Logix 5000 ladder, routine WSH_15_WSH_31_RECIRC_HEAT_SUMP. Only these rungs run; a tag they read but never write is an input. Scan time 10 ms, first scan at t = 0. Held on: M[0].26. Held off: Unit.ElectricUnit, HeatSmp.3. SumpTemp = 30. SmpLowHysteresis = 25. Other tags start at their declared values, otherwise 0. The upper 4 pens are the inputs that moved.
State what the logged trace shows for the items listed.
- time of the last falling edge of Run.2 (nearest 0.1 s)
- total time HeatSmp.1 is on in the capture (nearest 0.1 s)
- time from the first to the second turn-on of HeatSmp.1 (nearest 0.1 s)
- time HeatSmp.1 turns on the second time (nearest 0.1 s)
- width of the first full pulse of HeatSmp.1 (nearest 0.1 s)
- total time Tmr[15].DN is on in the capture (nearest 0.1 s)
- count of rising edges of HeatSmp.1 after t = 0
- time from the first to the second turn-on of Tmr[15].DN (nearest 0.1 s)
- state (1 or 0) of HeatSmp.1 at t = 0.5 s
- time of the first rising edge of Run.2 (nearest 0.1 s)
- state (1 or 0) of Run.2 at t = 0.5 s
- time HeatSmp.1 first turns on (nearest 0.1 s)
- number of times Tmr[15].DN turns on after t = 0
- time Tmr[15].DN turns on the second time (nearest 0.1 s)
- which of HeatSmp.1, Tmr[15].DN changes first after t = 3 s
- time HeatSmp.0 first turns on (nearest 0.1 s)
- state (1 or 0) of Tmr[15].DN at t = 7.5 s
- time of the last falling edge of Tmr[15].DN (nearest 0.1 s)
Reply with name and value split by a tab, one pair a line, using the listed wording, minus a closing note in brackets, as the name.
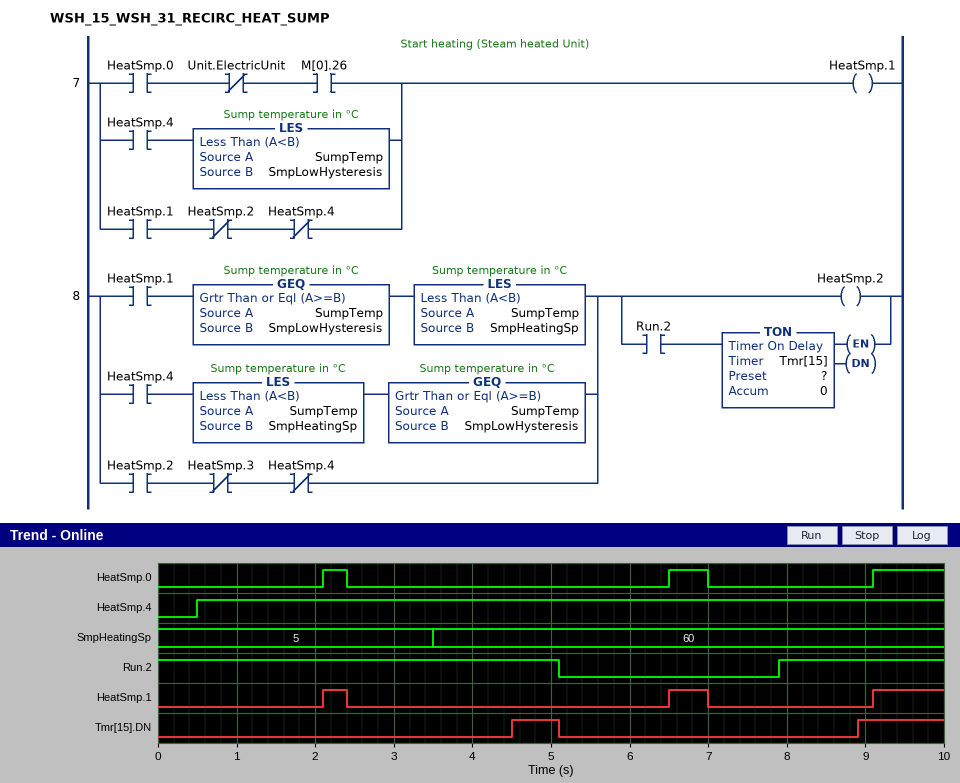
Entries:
time of the last falling edge of Run.2	5.1 s
total time HeatSmp.1 is on in the capture	1.7 s
time from the first to the second turn-on of HeatSmp.1	4.4 s
time HeatSmp.1 turns on the second time	6.5 s
width of the first full pulse of HeatSmp.1	0.3 s
total time Tmr[15].DN is on in the capture	1.7 s
count of rising edges of HeatSmp.1 after t = 0	3
time from the first to the second turn-on of Tmr[15].DN	4.4 s
state (1 or 0) of HeatSmp.1 at t = 0.5 s	0
time of the first rising edge of Run.2	7.9 s
state (1 or 0) of Run.2 at t = 0.5 s	1
time HeatSmp.1 first turns on	2.1 s
number of times Tmr[15].DN turns on after t = 0	2
time Tmr[15].DN turns on the second time	8.9 s
which of HeatSmp.1, Tmr[15].DN changes first after t = 3 s	Tmr[15].DN
time HeatSmp.0 first turns on	2.1 s
state (1 or 0) of Tmr[15].DN at t = 7.5 s	0
time of the last falling edge of Tmr[15].DN	5.1 s
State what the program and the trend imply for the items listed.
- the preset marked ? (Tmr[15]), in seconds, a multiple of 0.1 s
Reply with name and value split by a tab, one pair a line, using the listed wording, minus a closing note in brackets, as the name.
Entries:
the preset marked ? (Tmr[15]), in seconds, a multiple of 0.1 s	1.0 s
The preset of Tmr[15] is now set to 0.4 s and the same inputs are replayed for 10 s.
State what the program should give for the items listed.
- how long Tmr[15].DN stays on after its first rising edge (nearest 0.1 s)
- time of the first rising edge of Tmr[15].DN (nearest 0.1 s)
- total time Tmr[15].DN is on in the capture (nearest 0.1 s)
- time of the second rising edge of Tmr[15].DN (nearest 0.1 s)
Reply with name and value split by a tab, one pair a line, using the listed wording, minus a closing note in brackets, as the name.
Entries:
how long Tmr[15].DN stays on after its first rising edge	1.2 s
time of the first rising edge of Tmr[15].DN	3.9 s
total time Tmr[15].DN is on in the capture	2.9 s
time of the second rising edge of Tmr[15].DN	8.3 s
